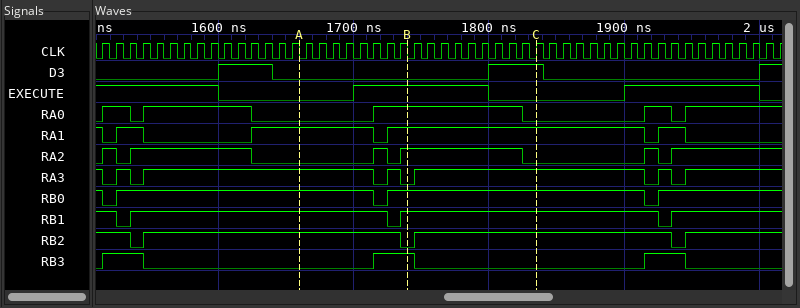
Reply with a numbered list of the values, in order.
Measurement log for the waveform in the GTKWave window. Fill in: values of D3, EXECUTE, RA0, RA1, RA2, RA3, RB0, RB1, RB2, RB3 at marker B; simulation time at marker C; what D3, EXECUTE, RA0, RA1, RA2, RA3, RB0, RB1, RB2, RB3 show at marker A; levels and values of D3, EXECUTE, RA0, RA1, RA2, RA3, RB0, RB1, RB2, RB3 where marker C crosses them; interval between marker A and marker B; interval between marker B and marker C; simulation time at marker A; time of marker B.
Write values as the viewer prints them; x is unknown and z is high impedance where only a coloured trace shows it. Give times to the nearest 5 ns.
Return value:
1. D3=0, EXECUTE=1, RA0=1, RA1=1, RA2=1, RA3=0, RB0=1, RB1=1, RB2=0, RB3=1
2. 1835 ns
3. D3=0, EXECUTE=0, RA0=0, RA1=1, RA2=0, RA3=1, RB0=1, RB1=1, RB2=1, RB3=0
4. D3=1, EXECUTE=0, RA0=0, RA1=1, RA2=0, RA3=1, RB0=1, RB1=1, RB2=1, RB3=0
5. 80 ns
6. 95 ns
7. 1660 ns
8. 1740 ns
